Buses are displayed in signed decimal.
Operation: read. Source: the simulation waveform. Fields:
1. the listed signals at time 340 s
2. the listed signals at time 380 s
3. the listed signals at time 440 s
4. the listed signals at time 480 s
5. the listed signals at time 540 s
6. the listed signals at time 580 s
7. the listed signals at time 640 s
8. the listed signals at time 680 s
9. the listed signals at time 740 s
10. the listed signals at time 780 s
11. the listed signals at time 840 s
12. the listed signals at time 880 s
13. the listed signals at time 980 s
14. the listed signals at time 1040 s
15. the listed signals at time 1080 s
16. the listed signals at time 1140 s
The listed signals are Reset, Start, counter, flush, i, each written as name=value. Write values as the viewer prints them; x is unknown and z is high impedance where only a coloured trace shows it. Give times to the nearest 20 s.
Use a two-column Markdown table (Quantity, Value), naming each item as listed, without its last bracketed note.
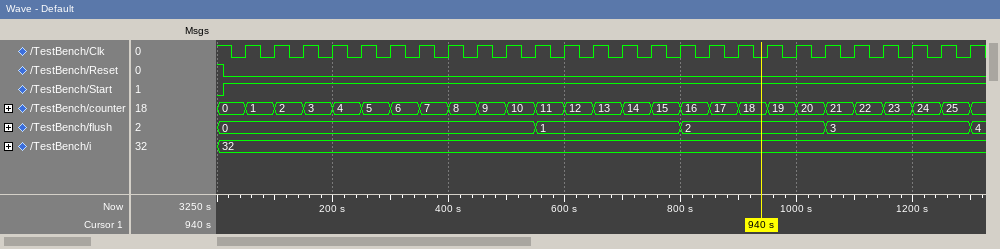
| Quantity | Value |
|---|---|
| the listed signals at time 340 s | Reset=0, Start=1, counter=6, flush=0, i=32 |
| the listed signals at time 380 s | Reset=0, Start=1, counter=7, flush=0, i=32 |
| the listed signals at time 440 s | Reset=0, Start=1, counter=8, flush=0, i=32 |
| the listed signals at time 480 s | Reset=0, Start=1, counter=9, flush=0, i=32 |
| the listed signals at time 540 s | Reset=0, Start=1, counter=10, flush=0, i=32 |
| the listed signals at time 580 s | Reset=0, Start=1, counter=11, flush=1, i=32 |
| the listed signals at time 640 s | Reset=0, Start=1, counter=12, flush=1, i=32 |
| the listed signals at time 680 s | Reset=0, Start=1, counter=13, flush=1, i=32 |
| the listed signals at time 740 s | Reset=0, Start=1, counter=14, flush=1, i=32 |
| the listed signals at time 780 s | Reset=0, Start=1, counter=15, flush=1, i=32 |
| the listed signals at time 840 s | Reset=0, Start=1, counter=16, flush=2, i=32 |
| the listed signals at time 880 s | Reset=0, Start=1, counter=17, flush=2, i=32 |
| the listed signals at time 980 s | Reset=0, Start=1, counter=19, flush=2, i=32 |
| the listed signals at time 1040 s | Reset=0, Start=1, counter=20, flush=2, i=32 |
| the listed signals at time 1080 s | Reset=0, Start=1, counter=21, flush=3, i=32 |
| the listed signals at time 1140 s | Reset=0, Start=1, counter=22, flush=3, i=32 |
